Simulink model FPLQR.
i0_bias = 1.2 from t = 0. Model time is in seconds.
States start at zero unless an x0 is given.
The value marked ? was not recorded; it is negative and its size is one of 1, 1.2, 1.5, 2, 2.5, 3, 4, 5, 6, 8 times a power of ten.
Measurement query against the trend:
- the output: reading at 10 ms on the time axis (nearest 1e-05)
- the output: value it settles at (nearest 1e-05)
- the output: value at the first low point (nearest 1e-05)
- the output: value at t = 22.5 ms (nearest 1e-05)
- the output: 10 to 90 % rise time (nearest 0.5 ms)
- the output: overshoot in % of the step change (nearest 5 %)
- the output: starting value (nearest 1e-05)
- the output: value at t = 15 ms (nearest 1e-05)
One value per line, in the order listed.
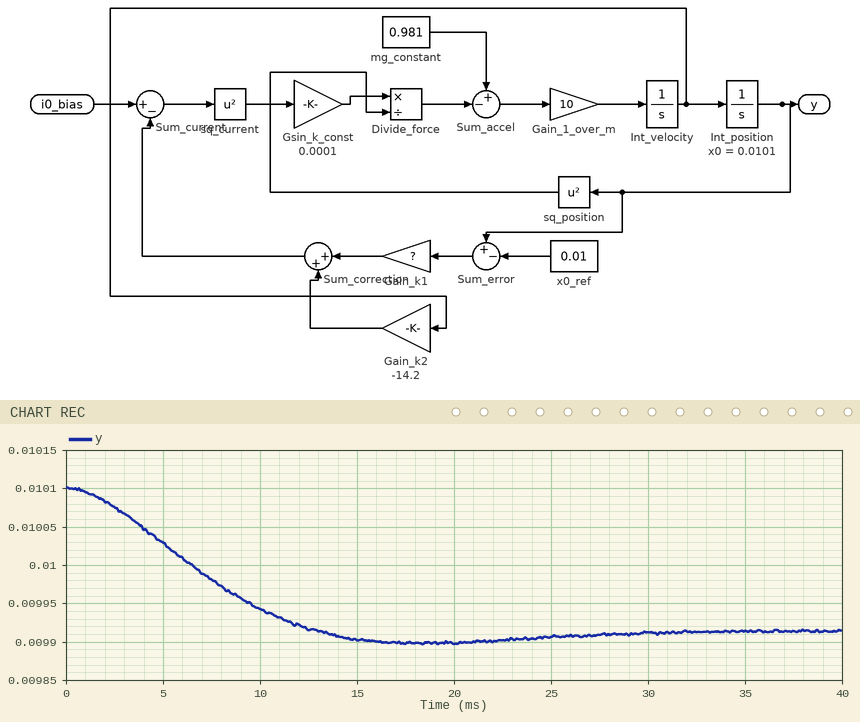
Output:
0.00994
0.00991
0.00990
0.00990
9.0 ms
10 %
0.01010
0.00990
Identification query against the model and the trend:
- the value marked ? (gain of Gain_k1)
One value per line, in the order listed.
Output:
-2500
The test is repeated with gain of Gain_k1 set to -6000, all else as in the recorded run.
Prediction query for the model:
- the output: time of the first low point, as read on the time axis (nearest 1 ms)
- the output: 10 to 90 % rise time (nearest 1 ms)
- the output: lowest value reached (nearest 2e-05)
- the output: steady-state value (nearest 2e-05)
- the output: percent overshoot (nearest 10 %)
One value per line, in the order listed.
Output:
10 ms
4 ms
0.00992
0.00996
30 %
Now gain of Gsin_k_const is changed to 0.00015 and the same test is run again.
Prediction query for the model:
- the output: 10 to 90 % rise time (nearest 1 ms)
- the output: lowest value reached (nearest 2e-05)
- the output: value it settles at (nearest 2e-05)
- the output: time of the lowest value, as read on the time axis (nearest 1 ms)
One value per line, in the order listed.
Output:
9 ms
0.00982
0.00984
18 ms
